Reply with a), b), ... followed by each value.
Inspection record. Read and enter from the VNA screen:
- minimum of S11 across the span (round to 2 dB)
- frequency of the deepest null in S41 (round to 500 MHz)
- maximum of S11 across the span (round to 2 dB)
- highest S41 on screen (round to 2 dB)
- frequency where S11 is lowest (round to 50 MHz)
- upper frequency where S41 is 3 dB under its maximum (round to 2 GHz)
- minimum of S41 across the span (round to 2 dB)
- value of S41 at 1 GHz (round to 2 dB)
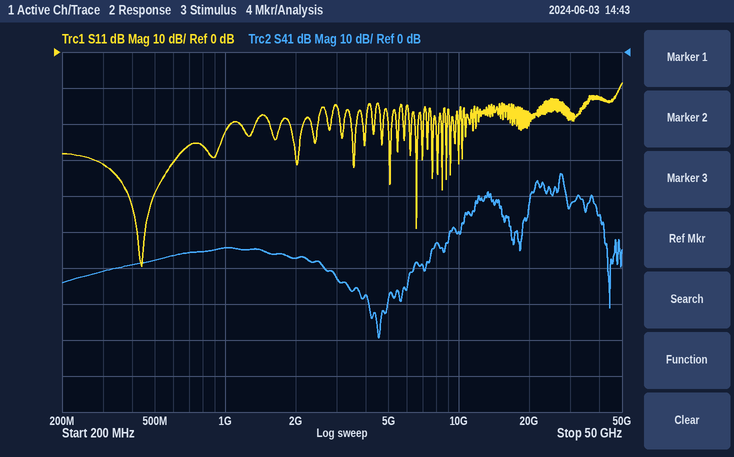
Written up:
a) -60 dB
b) 4.5 GHz
c) -8 dB
d) -34 dB
e) 450 MHz
f) 28 GHz
g) -80 dB
h) -54 dB
